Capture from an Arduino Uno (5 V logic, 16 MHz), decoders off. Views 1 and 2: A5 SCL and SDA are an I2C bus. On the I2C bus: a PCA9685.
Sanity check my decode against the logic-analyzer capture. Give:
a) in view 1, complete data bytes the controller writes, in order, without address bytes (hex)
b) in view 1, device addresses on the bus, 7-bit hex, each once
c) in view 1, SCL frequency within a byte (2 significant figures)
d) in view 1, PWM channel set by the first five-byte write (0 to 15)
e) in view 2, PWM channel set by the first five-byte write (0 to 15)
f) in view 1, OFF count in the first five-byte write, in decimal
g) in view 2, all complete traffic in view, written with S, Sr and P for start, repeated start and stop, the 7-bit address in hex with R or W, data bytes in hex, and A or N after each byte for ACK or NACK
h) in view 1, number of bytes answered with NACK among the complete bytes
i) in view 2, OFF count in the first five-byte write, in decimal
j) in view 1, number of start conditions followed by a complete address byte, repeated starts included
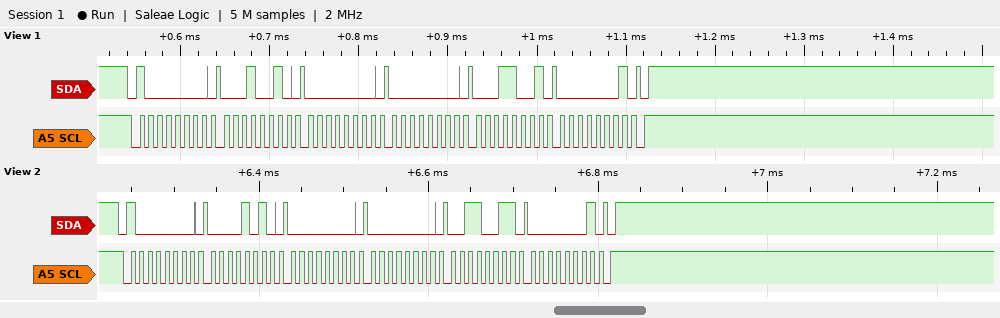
12 00 00 19 01
0x40
100 kHz
3
1
281
S 40W A 0A A 00 A 00 A 33 A 01 A P
0
307
1
